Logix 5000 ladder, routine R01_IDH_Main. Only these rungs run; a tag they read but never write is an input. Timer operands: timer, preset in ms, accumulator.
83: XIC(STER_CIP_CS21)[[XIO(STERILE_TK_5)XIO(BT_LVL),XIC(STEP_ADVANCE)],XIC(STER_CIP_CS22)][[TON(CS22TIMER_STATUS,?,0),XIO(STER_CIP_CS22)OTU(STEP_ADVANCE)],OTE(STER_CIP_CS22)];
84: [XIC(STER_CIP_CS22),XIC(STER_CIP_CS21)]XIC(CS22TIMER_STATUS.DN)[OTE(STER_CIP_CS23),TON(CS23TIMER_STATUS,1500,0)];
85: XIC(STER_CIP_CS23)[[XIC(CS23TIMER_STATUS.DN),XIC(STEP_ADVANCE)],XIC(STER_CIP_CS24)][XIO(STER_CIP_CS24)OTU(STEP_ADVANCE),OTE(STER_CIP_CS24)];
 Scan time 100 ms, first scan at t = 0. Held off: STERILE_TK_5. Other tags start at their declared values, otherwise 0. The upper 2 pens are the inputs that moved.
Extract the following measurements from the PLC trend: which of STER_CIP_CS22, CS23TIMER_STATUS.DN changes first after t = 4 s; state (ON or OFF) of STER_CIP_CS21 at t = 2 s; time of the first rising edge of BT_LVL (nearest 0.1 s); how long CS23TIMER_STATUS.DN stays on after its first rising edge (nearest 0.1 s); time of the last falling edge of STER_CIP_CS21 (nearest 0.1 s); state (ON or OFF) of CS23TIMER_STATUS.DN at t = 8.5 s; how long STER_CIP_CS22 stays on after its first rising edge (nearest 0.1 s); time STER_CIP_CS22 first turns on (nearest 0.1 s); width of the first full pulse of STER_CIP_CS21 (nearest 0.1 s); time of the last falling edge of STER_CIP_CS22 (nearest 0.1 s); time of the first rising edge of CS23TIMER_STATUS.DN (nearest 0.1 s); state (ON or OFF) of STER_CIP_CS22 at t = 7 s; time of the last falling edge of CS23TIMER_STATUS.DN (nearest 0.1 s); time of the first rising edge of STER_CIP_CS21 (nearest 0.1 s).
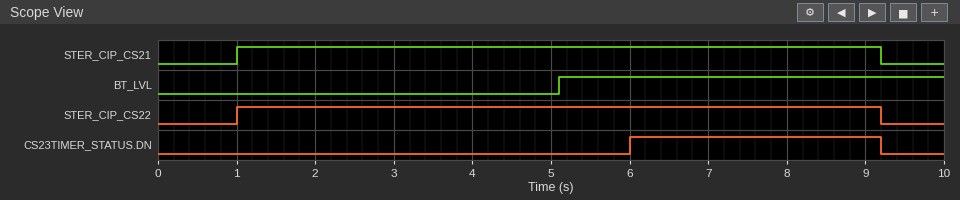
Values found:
CS23TIMER_STATUS.DN
ON
5.1 s
3.2 s
9.2 s
ON
8.2 s
1.0 s
8.2 s
9.2 s
6.0 s
ON
9.2 s
1.0 s
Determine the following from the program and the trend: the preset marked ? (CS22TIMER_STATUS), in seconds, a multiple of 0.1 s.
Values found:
3.5 s
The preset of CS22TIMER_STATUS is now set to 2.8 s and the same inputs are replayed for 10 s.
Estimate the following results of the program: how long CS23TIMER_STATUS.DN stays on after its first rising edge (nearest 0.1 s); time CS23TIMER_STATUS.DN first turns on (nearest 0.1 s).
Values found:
3.9 s
5.3 s
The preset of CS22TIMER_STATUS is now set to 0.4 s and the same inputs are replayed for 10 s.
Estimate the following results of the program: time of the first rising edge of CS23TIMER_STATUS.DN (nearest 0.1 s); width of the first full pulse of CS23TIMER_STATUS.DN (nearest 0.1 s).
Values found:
2.9 s
6.3 s
